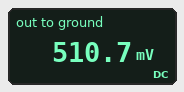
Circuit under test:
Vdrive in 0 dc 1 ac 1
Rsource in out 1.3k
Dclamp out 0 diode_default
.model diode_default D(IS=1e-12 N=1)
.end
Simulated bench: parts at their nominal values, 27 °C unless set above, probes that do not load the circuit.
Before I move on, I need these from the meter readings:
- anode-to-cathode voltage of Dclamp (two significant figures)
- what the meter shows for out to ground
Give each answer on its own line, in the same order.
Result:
510 mV
510.7 mV
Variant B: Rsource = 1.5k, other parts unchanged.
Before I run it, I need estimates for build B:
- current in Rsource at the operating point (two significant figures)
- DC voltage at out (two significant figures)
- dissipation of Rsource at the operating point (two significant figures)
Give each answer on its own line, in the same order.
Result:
330 µA
510 mV
160 µW
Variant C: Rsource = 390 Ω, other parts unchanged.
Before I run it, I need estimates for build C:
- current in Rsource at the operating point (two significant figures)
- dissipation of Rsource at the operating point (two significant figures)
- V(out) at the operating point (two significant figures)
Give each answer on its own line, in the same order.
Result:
1.2 mA
540 µW
540 mV
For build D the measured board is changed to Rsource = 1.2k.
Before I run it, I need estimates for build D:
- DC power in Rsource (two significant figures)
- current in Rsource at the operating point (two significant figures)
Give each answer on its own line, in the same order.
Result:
200 µW
410 µA
